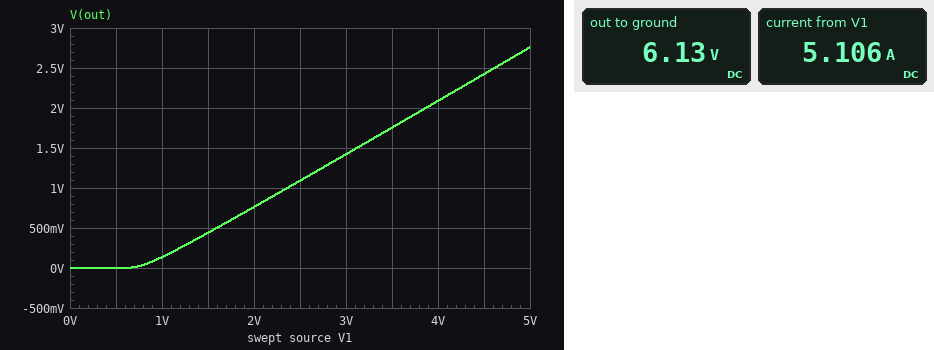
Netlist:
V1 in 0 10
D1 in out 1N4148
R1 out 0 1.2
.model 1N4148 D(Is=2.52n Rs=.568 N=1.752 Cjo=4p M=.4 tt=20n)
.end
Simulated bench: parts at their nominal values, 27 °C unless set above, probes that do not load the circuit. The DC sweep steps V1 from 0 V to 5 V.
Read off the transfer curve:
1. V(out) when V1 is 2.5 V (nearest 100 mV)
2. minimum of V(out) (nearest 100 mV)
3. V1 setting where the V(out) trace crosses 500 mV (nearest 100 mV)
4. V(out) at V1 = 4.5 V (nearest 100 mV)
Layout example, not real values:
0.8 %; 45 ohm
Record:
1.1 V; 0 V; 1.6 V; 2.4 V
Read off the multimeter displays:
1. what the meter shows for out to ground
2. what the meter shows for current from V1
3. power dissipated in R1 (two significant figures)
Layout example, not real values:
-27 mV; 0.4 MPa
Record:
6.13 V; 5.106 A; 31 W
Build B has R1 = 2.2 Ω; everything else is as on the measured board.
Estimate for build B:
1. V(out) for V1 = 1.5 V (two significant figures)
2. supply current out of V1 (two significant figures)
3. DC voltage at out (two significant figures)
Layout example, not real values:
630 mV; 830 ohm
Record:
530 mV; 3.3 A; 7.2 V
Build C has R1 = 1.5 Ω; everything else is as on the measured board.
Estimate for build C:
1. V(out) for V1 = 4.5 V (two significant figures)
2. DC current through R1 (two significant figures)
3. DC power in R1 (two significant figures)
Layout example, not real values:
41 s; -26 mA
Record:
2.6 V; 4.4 A; 29 W
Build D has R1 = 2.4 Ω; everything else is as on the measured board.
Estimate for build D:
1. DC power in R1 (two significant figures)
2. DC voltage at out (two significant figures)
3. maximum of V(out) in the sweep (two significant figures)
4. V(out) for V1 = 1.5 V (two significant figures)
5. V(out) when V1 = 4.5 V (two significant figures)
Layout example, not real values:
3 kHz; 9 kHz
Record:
22 W; 7.3 V; 3.3 V; 540 mV; 2.9 V
